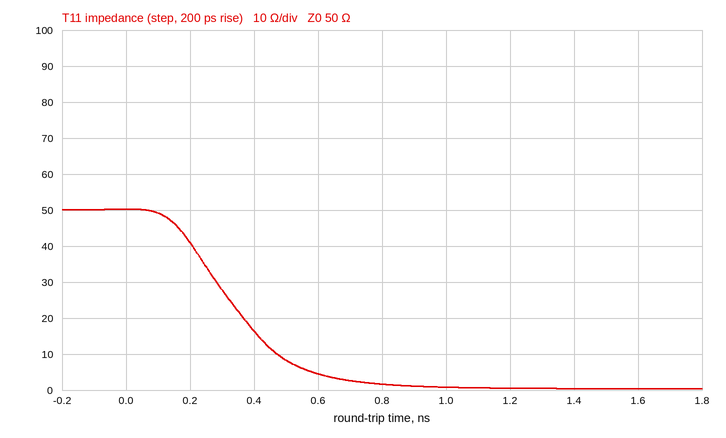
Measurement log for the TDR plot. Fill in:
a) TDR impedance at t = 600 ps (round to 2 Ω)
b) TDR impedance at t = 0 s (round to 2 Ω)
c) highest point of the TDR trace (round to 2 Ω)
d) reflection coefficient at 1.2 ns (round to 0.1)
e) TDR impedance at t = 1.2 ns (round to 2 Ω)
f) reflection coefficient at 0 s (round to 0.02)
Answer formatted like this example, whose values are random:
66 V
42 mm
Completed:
4 Ω
50 Ω
50 Ω
-1.0
0 Ω
0.00
